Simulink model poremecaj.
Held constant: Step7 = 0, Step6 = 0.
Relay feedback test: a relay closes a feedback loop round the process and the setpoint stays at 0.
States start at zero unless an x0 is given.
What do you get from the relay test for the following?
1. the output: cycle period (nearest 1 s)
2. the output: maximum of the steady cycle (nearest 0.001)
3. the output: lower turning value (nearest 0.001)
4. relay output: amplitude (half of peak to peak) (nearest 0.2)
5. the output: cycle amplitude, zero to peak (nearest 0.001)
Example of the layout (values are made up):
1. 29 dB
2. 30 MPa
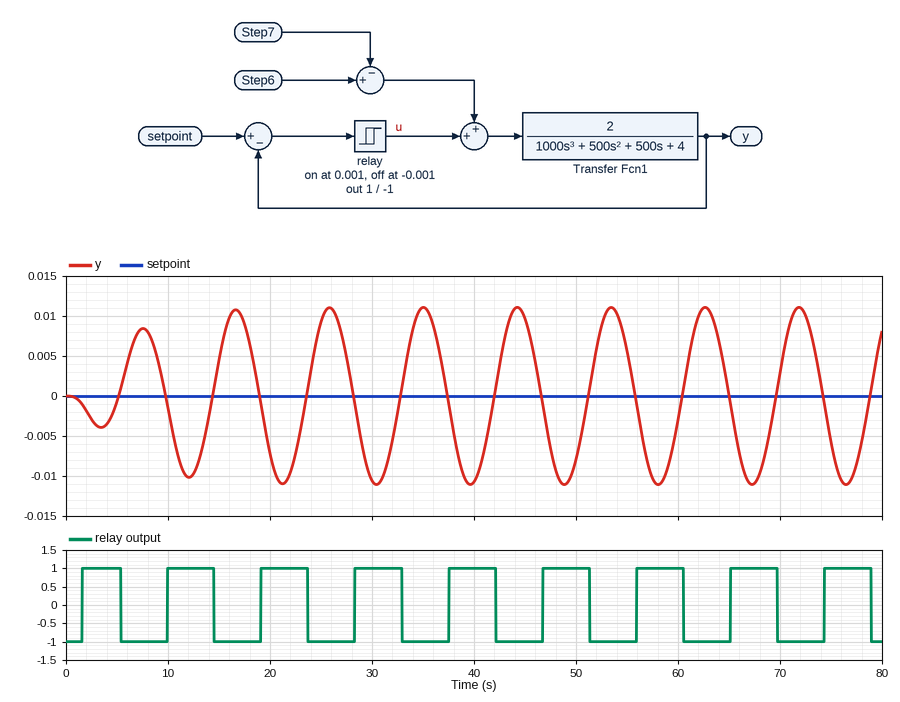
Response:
1. 9 s
2. 0.011
3. -0.011
4. 1.0
5. 0.011
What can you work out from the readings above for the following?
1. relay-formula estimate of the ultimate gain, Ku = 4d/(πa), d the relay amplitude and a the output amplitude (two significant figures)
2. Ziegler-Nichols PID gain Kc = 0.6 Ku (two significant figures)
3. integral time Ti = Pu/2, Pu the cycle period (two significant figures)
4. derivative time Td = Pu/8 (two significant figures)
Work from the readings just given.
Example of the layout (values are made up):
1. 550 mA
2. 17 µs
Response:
1. 120
2. 72
3. 4.5 s
4. 1.1 s
